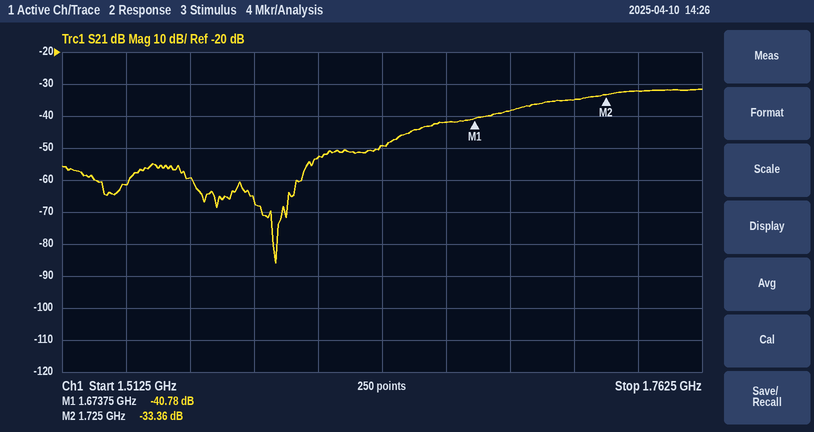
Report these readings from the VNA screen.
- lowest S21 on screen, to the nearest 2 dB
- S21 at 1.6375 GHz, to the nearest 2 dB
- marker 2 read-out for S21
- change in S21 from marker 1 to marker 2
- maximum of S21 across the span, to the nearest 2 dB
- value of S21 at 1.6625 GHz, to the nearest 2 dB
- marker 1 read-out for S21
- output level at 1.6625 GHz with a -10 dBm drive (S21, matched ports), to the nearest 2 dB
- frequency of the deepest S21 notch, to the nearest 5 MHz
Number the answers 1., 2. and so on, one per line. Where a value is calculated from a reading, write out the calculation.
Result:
1. -86 dB
2. -50 dB
3. -33.36 dB
4. -33.36 − (-40.78) = 7.42 dB
5. -32 dB
6. -42 dB
7. -40.78 dB
8. -10 dBm + (-42 dB) = -52 dBm
9. 1.595 GHz
